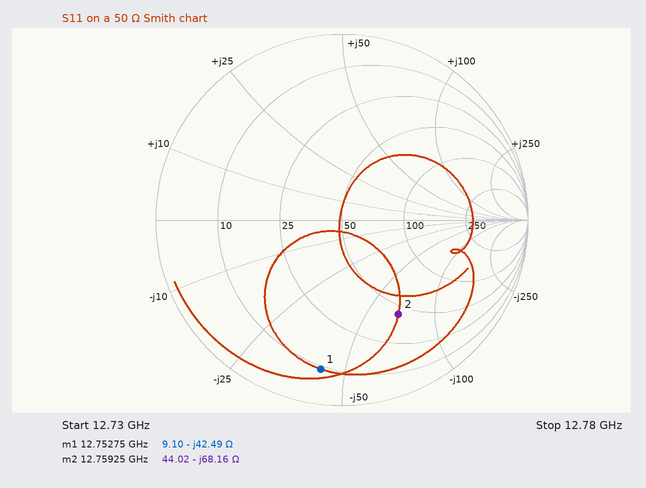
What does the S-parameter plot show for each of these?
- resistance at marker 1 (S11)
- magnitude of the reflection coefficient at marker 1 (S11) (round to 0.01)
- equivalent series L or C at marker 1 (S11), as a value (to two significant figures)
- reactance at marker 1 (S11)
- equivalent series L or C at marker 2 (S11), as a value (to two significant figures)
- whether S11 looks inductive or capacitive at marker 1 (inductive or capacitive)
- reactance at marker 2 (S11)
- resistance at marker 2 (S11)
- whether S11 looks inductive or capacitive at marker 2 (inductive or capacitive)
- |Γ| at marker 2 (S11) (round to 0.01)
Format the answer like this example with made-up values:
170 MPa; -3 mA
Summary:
9.10 Ω; 0.81; 290 fF; -42.49 Ω; 180 fF; capacitive; -68.16 Ω; 44.02 Ω; capacitive; 0.59
